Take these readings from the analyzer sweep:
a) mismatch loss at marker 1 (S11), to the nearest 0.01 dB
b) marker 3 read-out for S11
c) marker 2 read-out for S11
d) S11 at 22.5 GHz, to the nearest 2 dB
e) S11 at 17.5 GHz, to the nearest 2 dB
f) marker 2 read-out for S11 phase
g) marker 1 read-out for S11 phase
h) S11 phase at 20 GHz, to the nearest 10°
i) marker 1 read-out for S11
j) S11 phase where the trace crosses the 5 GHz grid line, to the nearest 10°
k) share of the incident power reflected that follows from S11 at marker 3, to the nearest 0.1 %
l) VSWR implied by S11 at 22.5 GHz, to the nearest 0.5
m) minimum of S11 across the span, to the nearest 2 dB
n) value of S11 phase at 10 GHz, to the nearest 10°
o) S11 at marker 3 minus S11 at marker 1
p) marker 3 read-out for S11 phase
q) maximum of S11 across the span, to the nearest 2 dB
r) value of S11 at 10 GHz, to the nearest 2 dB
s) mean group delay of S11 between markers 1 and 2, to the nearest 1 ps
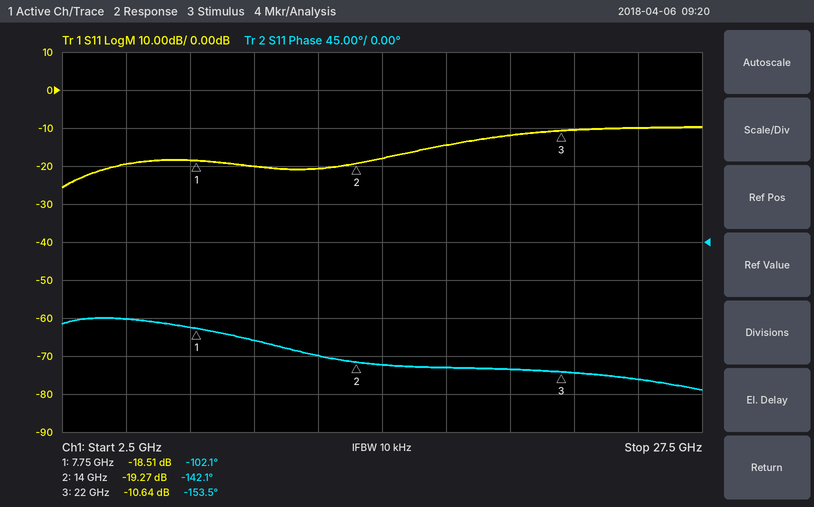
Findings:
0.06 dB
-10.64 dB
-19.27 dB
-10 dB
-14 dB
-142.1°
-102.1°
-150°
-18.51 dB
-90°
8.6 %
2.0
-26 dB
-120°
7.87 dB
-153.5°
-10 dB
-20 dB
18 ps
